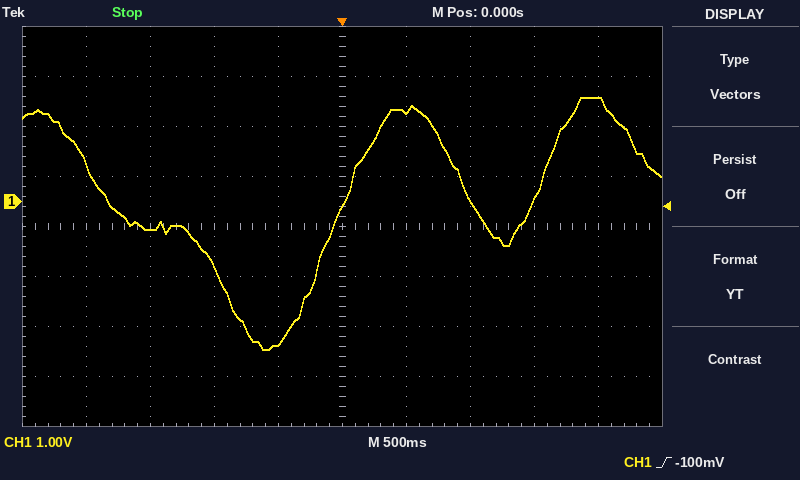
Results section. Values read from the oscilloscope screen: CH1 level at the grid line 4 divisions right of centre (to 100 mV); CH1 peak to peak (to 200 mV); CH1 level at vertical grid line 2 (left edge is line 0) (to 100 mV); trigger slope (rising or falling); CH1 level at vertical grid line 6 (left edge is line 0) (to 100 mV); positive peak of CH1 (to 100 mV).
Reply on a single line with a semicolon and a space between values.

2.1 V; 5.0 V; -600 mV; rising; 1.8 V; 2.1 V
